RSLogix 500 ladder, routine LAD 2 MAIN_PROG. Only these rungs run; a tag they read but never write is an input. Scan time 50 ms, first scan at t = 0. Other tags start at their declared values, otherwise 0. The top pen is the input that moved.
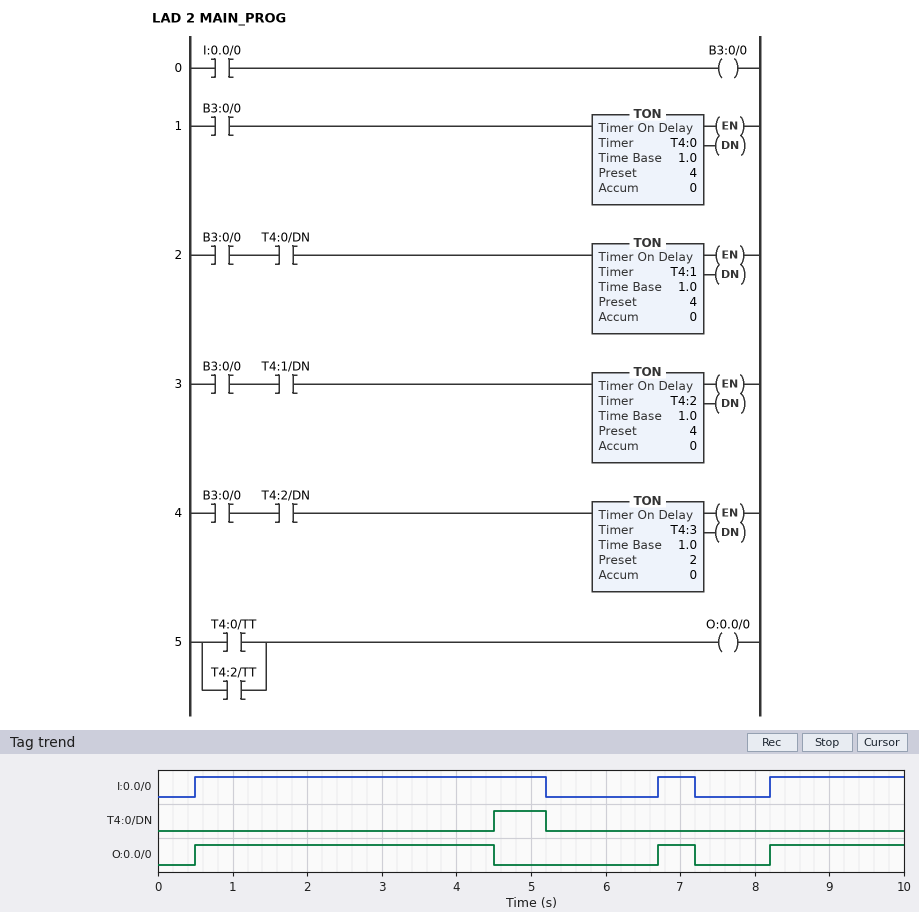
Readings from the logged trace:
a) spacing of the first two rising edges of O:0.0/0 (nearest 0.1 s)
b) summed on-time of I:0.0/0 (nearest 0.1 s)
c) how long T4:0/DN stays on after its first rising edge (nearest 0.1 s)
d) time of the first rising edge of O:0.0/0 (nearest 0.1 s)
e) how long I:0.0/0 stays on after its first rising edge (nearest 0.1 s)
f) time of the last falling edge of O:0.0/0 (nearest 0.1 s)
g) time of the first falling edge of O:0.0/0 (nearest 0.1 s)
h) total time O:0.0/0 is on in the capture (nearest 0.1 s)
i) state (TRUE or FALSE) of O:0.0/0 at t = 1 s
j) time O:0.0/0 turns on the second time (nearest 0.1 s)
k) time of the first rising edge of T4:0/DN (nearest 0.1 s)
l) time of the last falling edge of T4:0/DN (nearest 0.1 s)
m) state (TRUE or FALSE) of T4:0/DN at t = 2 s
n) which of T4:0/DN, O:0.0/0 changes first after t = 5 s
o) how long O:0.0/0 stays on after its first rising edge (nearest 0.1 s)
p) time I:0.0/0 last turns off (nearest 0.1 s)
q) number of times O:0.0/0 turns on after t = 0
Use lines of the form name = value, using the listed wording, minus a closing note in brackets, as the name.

spacing of the first two rising edges of O:0.0/0 = 6.2 s
summed on-time of I:0.0/0 = 7.0 s
how long T4:0/DN stays on after its first rising edge = 0.7 s
time of the first rising edge of O:0.0/0 = 0.5 s
how long I:0.0/0 stays on after its first rising edge = 4.7 s
time of the last falling edge of O:0.0/0 = 7.2 s
time of the first falling edge of O:0.0/0 = 4.5 s
total time O:0.0/0 is on in the capture = 6.3 s
state (TRUE or FALSE) of O:0.0/0 at t = 1 s = TRUE
time O:0.0/0 turns on the second time = 6.7 s
time of the first rising edge of T4:0/DN = 4.5 s
time of the last falling edge of T4:0/DN = 5.2 s
state (TRUE or FALSE) of T4:0/DN at t = 2 s = FALSE
which of T4:0/DN, O:0.0/0 changes first after t = 5 s = T4:0/DN
how long O:0.0/0 stays on after its first rising edge = 4.0 s
time I:0.0/0 last turns off = 7.2 s
number of times O:0.0/0 turns on after t = 0 = 3
